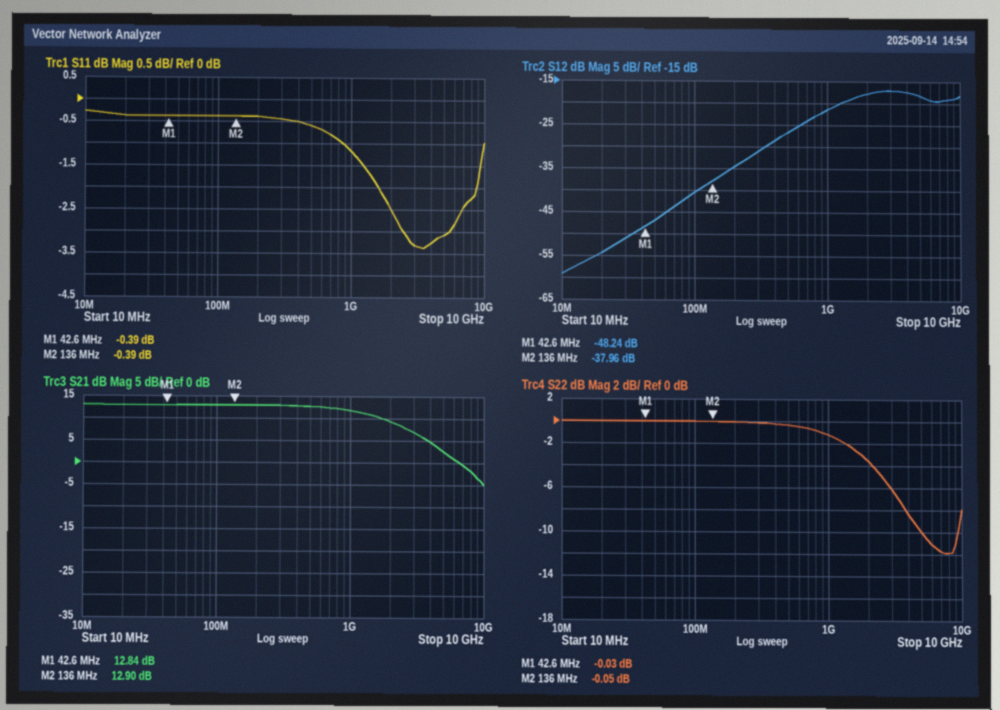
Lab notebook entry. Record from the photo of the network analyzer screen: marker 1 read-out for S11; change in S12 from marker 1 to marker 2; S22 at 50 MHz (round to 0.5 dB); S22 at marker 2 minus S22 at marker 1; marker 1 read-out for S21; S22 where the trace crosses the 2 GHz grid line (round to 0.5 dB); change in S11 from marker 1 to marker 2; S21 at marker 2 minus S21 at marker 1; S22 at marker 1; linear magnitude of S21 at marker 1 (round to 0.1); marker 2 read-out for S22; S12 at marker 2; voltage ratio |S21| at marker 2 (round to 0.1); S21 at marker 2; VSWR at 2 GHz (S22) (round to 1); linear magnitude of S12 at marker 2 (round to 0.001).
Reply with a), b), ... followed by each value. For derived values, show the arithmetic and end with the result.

a) -0.39 dB
b) -37.96 − (-48.24) = 10.28 dB
c) 0.0 dB
d) -0.05 − (-0.03) = -0.02 dB
e) 12.84 dB
f) -3.5 dB
g) -0.39 − (-0.39) = 0.00 dB
h) 12.9 − (12.84) = 0.06 dB
i) -0.03 dB
j) 10^(12.84/20) ≈ 4.4
k) -0.05 dB
l) -37.96 dB
m) 10^(12.9/20) ≈ 4.4
n) 12.90 dB
o) |Γ| = 10^(-3.5/20) = 0.6683; VSWR = (1 + 0.6683)/(1 − 0.6683) ≈ 5
p) 10^(-37.96/20) ≈ 0.013
